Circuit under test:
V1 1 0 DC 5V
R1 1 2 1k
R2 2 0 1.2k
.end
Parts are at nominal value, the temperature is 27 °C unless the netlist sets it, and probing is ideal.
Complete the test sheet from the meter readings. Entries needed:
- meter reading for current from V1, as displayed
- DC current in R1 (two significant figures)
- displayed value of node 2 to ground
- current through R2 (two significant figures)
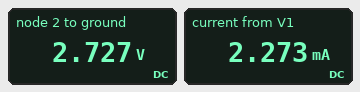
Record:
2.273 mA
2.3 mA
2.727 V
2.3 mA
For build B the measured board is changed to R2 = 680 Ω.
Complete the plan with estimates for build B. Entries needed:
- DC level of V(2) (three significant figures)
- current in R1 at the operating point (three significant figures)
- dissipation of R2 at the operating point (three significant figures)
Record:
2.02 V
2.98 mA
6.02 mW
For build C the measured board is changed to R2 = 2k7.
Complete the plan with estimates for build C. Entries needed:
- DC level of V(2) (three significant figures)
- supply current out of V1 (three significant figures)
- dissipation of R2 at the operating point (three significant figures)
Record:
3.65 V
1.35 mA
4.93 mW
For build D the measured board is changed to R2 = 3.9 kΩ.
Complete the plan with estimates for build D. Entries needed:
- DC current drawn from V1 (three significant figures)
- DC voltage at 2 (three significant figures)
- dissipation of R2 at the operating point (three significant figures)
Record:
1.02 mA
3.98 V
4.06 mW
